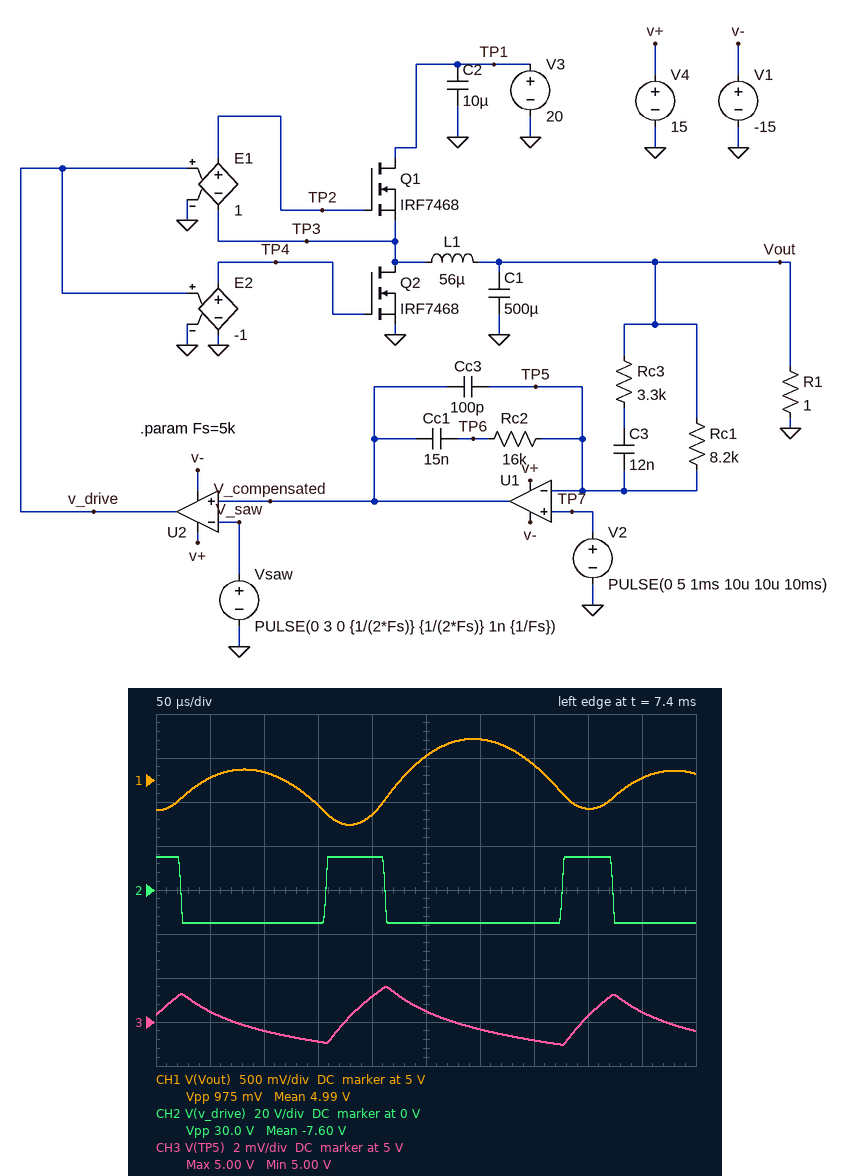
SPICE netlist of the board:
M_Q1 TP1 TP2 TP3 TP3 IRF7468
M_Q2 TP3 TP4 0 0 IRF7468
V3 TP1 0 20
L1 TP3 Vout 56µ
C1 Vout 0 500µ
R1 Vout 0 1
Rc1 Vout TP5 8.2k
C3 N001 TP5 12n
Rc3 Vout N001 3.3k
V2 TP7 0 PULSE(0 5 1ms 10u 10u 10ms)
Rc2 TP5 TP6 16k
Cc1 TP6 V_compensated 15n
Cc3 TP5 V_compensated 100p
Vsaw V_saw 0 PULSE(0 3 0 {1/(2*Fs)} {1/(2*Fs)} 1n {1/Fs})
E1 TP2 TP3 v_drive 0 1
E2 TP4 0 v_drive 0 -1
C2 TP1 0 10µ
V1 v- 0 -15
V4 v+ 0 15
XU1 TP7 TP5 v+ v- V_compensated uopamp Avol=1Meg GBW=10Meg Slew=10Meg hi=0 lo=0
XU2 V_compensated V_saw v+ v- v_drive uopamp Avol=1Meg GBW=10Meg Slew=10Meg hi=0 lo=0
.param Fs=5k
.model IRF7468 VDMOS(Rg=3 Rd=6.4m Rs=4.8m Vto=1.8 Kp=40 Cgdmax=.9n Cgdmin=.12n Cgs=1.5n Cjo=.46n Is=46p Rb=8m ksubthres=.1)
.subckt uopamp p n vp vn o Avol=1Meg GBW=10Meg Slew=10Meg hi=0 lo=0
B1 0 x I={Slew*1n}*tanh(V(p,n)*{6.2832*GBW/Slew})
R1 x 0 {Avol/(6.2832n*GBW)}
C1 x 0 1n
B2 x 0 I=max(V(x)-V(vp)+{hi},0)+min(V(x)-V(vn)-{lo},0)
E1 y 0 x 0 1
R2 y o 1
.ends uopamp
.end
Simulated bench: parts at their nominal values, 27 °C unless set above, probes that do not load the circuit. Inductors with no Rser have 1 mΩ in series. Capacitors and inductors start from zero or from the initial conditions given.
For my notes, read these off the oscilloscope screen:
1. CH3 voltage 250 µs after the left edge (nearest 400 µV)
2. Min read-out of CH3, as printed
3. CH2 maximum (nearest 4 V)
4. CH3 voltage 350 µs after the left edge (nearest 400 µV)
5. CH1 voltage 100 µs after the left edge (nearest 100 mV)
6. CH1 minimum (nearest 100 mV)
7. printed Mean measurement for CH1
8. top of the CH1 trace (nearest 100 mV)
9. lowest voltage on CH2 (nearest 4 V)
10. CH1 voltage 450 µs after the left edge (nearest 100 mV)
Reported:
5.0004 V
5.00 V
16 V
4.9992 V
5.1 V
4.5 V
4.99 V
5.5 V
-16 V
5.0 V
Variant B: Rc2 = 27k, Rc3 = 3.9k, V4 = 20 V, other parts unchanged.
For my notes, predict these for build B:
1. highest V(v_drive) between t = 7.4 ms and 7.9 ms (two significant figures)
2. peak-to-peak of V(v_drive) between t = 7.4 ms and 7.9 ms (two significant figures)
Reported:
20 V
35 V
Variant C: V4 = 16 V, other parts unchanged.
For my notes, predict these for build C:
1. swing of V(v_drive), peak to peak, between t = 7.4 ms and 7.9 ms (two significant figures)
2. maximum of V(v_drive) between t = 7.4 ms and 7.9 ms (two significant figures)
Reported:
31 V
16 V
